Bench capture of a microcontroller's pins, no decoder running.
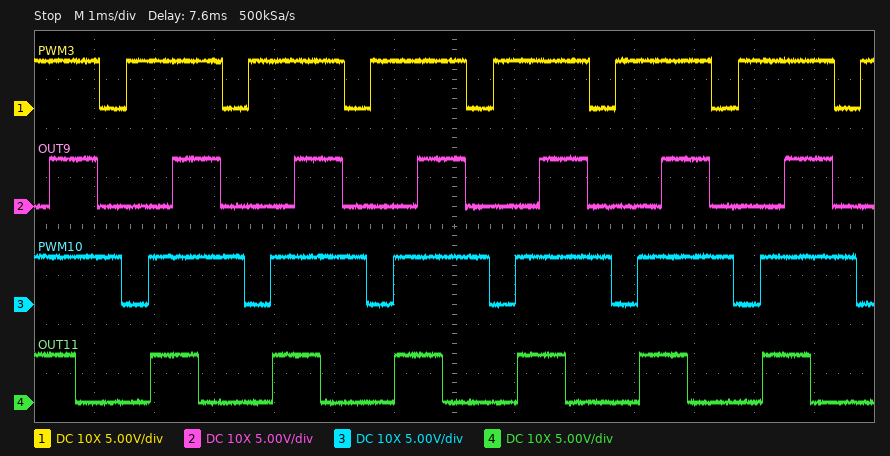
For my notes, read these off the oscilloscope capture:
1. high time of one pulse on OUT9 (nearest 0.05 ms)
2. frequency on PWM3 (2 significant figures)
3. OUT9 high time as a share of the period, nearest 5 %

0.80 ms
490 Hz
40 %
